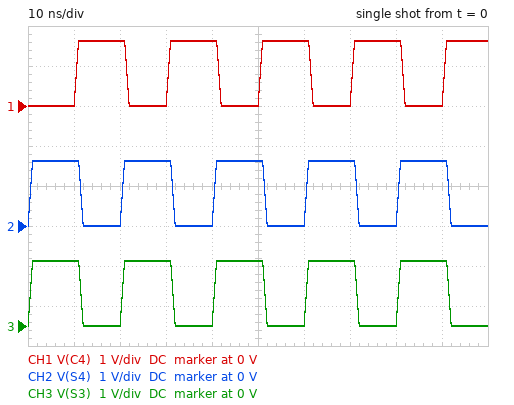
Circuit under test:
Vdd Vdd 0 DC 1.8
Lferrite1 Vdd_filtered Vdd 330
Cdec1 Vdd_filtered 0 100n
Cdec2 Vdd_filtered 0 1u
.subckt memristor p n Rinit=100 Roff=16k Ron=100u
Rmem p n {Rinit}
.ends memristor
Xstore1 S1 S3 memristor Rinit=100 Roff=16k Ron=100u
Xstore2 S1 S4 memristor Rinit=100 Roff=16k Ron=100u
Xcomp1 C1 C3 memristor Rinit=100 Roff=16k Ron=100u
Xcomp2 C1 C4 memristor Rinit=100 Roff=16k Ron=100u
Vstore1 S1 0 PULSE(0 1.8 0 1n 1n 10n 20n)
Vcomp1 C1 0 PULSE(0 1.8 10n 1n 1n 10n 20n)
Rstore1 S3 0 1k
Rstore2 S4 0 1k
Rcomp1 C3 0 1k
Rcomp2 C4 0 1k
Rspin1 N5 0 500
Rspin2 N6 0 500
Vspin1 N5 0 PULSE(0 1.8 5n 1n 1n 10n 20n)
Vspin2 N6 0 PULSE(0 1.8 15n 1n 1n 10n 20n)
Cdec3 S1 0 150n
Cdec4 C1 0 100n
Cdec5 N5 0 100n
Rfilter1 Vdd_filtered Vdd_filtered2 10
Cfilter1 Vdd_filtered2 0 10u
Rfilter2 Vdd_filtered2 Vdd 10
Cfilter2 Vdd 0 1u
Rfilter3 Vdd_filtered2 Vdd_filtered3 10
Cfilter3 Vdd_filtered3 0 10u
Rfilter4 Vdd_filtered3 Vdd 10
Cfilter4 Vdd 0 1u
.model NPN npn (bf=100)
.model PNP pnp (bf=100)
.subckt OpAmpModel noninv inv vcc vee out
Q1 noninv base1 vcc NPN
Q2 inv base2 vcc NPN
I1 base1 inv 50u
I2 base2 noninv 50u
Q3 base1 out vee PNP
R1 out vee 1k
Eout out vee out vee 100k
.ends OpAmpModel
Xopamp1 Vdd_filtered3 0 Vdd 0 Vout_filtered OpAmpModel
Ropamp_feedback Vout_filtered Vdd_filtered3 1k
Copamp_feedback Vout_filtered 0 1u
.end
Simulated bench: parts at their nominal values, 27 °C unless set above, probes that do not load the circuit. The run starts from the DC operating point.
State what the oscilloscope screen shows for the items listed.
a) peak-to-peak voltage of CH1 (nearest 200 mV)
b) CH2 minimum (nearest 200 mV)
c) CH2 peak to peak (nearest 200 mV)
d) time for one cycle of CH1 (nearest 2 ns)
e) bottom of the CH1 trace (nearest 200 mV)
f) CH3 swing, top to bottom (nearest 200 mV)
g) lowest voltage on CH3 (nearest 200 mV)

1.6 V
0 V
1.6 V
20 ns
0 V
1.6 V
0 V
